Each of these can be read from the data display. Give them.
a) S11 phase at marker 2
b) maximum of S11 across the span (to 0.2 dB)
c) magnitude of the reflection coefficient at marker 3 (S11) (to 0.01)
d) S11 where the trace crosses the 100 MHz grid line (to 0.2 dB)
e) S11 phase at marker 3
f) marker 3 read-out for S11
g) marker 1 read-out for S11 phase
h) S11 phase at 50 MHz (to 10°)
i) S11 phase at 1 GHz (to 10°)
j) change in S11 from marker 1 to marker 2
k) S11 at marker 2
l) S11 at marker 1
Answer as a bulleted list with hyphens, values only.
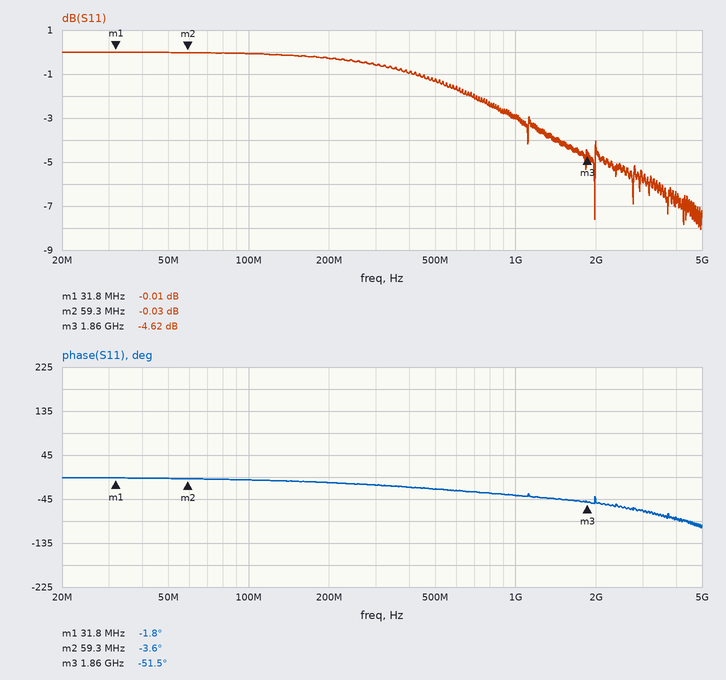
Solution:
- -3.6°
- 0.0 dB
- 0.59
- 0.0 dB
- -51.5°
- -4.62 dB
- -1.8°
- 0°
- -40°
- -0.02 dB
- -0.03 dB
- -0.01 dB
